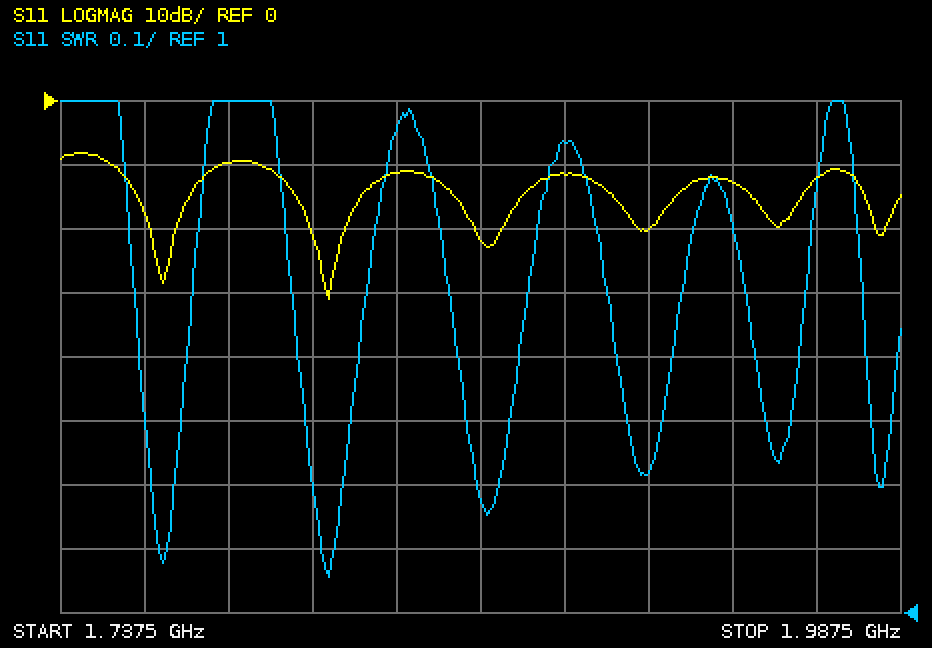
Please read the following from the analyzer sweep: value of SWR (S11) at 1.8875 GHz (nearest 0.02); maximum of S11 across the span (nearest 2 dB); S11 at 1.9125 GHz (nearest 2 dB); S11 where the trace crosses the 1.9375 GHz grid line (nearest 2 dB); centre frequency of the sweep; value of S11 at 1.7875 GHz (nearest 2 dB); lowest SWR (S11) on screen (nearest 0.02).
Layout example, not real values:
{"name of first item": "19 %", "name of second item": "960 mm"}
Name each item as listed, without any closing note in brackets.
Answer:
{"value of SWR (S11) at 1.8875 GHz": "1.74", "maximum of S11 across the span": "-8 dB", "S11 at 1.9125 GHz": "-20 dB", "S11 where the trace crosses the 1.9375 GHz grid line": "-12 dB", "centre frequency of the sweep": "1.8625 GHz", "value of S11 at 1.7875 GHz": "-10 dB", "lowest SWR (S11) on screen": "1.06"}
